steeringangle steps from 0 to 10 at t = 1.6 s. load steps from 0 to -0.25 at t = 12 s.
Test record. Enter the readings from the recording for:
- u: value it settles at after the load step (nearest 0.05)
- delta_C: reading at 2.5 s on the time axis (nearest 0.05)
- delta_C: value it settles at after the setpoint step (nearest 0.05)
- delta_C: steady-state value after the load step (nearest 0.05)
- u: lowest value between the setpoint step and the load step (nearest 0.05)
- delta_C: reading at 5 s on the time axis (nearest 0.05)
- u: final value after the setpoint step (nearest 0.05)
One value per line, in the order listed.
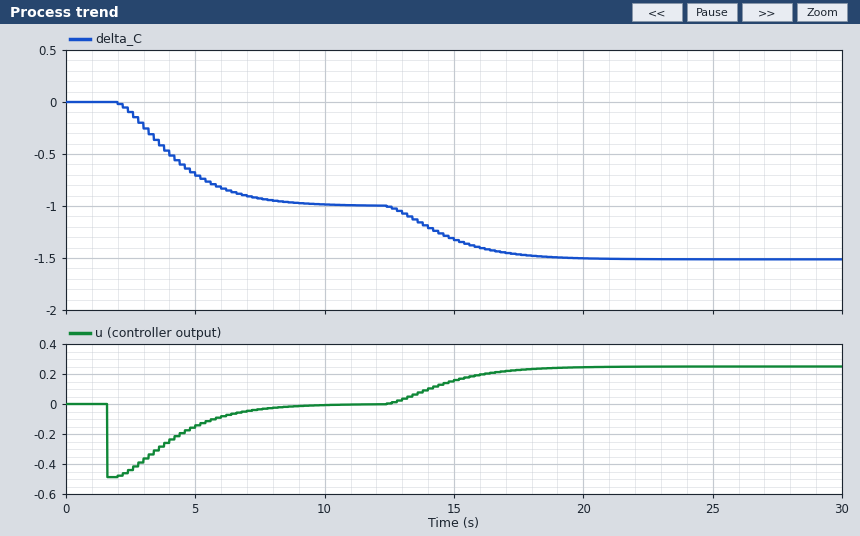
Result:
0.25
-0.10
-1.00
-1.50
-0.50
-0.70
0.00
